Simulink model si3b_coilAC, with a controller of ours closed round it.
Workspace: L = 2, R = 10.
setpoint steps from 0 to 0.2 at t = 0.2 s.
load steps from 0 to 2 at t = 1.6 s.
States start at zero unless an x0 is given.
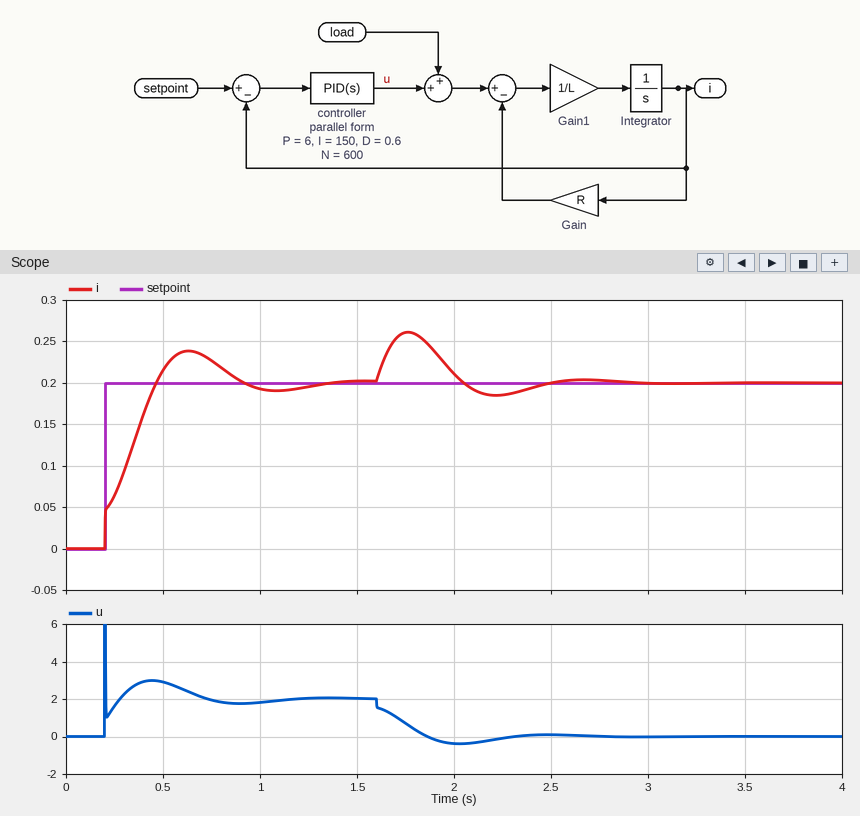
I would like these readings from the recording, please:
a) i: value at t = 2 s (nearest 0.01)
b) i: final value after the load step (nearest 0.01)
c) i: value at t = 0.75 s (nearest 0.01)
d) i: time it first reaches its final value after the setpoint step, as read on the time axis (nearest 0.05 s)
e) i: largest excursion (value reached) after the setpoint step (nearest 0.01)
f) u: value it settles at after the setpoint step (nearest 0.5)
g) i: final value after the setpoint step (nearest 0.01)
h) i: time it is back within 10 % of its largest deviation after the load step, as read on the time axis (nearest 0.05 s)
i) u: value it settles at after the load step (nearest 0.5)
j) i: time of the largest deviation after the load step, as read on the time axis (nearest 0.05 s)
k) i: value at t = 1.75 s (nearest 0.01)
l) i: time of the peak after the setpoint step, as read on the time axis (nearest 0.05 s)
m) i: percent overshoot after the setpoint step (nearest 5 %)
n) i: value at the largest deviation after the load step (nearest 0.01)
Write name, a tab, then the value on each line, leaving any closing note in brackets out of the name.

i: value at t = 2 s	0.21
i: final value after the load step	0.20
i: value at t = 0.75 s	0.23
i: time it first reaches its final value after the setpoint step, as read on the time axis	0.45 s
i: largest excursion (value reached) after the setpoint step	0.24
u: value it settles at after the setpoint step	2.0
i: final value after the setpoint step	0.20
i: time it is back within 10 % of its largest deviation after the load step, as read on the time axis	2.40 s
u: value it settles at after the load step	0.0
i: time of the largest deviation after the load step, as read on the time axis	1.75 s
i: value at t = 1.75 s	0.26
i: time of the peak after the setpoint step, as read on the time axis	0.65 s
i: percent overshoot after the setpoint step	20 %
i: value at the largest deviation after the load step	0.26
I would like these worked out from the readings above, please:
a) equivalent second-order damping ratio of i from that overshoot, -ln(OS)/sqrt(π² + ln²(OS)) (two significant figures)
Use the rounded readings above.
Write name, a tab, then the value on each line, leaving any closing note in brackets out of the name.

equivalent second-order damping ratio of i from that overshoot, -ln(OS)/sqrt(π² + ln²(OS))	0.46
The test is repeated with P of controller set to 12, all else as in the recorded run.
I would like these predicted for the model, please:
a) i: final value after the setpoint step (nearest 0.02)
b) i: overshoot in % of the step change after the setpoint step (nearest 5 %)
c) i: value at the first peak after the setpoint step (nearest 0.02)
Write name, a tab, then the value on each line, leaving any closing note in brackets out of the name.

i: final value after the setpoint step	0.20
i: overshoot in % of the step change after the setpoint step	10 %
i: value at the first peak after the setpoint step	0.22
